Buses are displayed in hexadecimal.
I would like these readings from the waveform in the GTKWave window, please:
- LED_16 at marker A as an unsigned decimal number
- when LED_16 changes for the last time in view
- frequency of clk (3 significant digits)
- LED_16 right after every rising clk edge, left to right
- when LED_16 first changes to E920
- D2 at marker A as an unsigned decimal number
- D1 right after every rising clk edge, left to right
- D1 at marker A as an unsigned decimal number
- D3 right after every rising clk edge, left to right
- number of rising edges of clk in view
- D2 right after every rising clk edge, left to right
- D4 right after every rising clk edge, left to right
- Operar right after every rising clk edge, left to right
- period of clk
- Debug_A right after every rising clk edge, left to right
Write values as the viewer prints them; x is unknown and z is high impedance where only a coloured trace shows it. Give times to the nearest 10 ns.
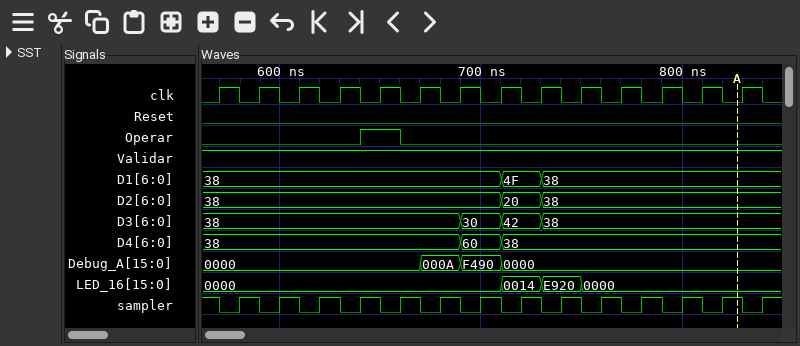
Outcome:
0
750 ns
50.0 MHz
0000, 0000, 0000, 0000, 0000, 0000, 0000, 0014, E920, 0000, 0000, 0000, 0000, 0000
730 ns
56
38, 38, 38, 38, 38, 38, 38, 4F, 38, 38, 38, 38, 38, 38
56
38, 38, 38, 38, 38, 38, 30, 42, 38, 38, 38, 38, 38, 38
14
38, 38, 38, 38, 38, 38, 38, 20, 38, 38, 38, 38, 38, 38
38, 38, 38, 38, 38, 38, 60, 38, 38, 38, 38, 38, 38, 38
0 0 0 0 1 0 0 0 0 0 0 0 0 0
20 ns
0000, 0000, 0000, 0000, 0000, 000A, F490, 0000, 0000, 0000, 0000, 0000, 0000, 0000
